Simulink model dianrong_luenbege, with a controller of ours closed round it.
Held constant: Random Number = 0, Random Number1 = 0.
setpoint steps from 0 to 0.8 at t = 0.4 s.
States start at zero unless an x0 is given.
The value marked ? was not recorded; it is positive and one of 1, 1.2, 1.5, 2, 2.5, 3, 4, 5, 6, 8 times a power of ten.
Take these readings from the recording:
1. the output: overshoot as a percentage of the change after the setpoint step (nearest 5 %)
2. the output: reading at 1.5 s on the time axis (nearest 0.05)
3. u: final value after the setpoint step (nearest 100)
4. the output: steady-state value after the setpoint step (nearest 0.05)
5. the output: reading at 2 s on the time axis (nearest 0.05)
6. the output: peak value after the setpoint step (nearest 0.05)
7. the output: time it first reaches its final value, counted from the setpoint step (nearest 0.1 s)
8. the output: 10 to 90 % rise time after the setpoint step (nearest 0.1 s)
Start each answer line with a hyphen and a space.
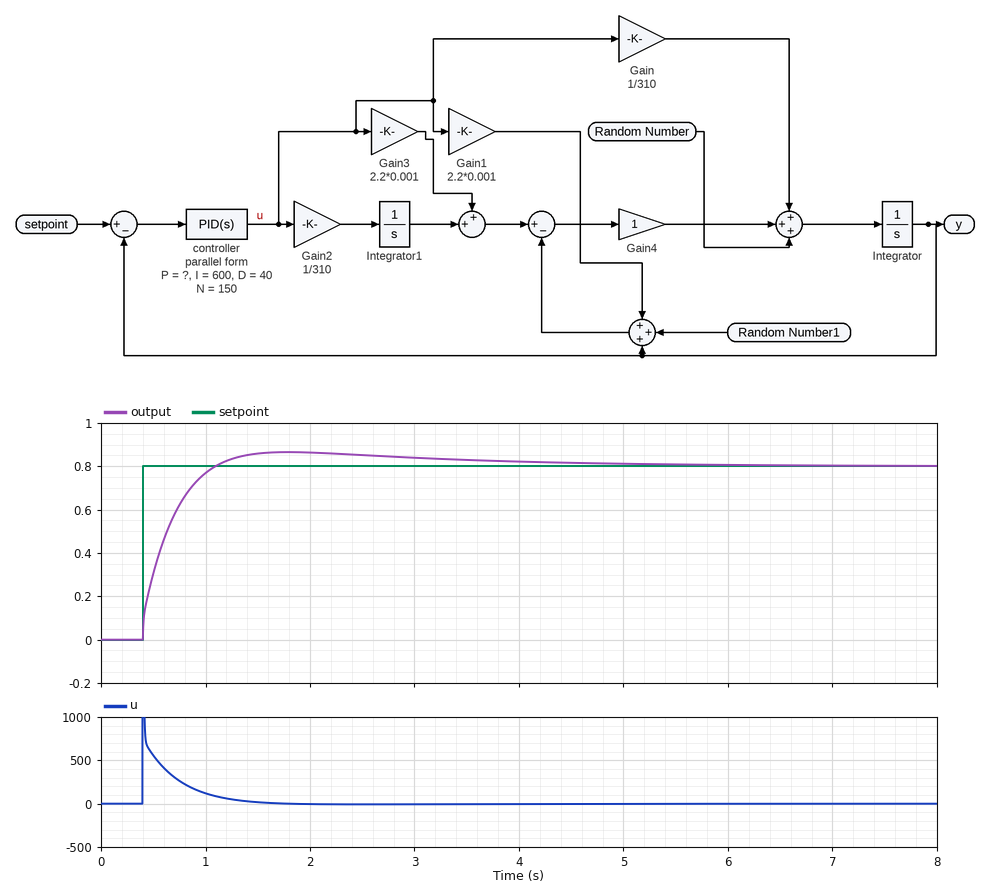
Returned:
- 10 %
- 0.85
- 0
- 0.80
- 0.85
- 0.85
- 0.7 s
- 0.5 s
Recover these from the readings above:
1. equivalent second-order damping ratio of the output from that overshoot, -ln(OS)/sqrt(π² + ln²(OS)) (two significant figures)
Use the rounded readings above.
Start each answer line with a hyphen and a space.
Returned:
- 0.59
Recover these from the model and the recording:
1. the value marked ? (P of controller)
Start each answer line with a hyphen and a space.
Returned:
- 1200
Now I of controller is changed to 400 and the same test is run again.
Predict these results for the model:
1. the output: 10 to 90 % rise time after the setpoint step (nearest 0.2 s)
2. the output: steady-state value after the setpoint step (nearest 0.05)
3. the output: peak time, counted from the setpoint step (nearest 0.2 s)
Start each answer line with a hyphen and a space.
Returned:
- 0.6 s
- 0.80
- 1.6 s
